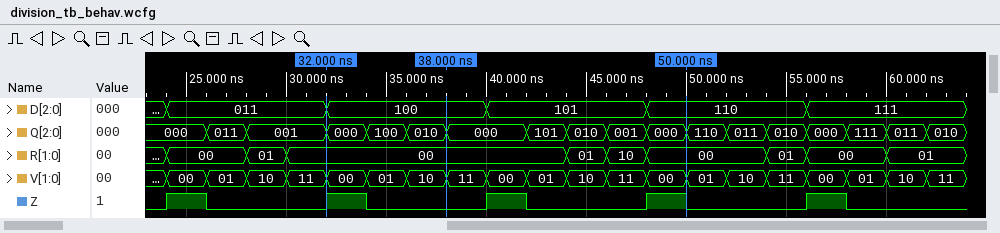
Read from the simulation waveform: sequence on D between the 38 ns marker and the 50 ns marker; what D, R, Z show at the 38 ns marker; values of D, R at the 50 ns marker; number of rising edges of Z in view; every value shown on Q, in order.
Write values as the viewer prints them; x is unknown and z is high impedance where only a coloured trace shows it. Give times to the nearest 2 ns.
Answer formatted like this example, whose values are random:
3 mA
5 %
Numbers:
100, 101, 110
D=100, R=00, Z=0
D=110, R=00
5
000, 011, 001, 000, 100, 010, 000, 101, 010, 001, 000, 110, 011, 010, 000, 111, 011, 010
